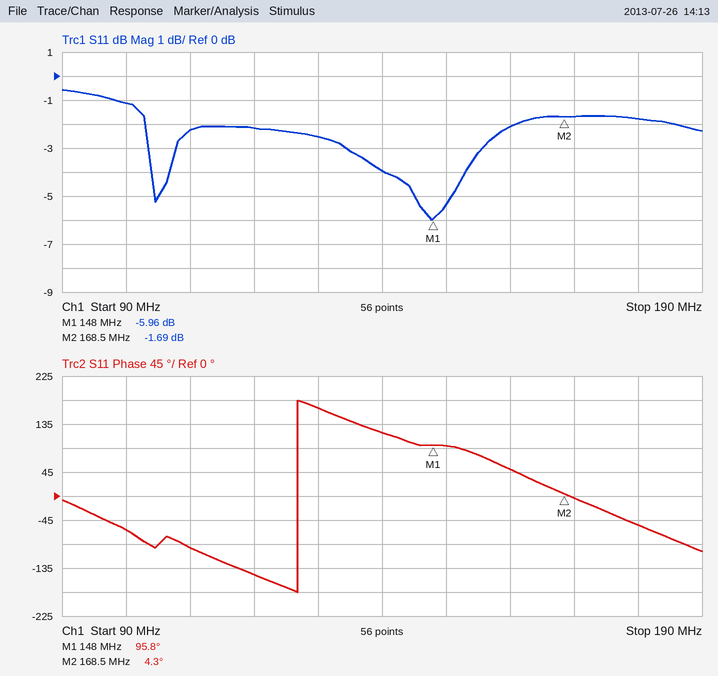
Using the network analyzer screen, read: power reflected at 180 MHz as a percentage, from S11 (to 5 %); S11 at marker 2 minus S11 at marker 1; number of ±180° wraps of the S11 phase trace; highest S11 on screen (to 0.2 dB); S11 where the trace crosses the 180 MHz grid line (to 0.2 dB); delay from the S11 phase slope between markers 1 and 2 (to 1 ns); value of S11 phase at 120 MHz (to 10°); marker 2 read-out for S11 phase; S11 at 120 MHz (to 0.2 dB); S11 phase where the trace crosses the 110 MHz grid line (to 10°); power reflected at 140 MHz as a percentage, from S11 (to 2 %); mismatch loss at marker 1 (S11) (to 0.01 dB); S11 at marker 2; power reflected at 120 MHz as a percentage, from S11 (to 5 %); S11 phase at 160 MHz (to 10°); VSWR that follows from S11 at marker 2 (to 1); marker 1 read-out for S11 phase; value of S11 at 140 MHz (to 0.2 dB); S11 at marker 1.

65 %
4.27 dB
1
-0.6 dB
-1.8 dB
12 ns
-150°
4.3°
-2.2 dB
-100°
40 %
1.27 dB
-1.69 dB
60 %
50°
10
95.8°
-4.0 dB
-5.96 dB
